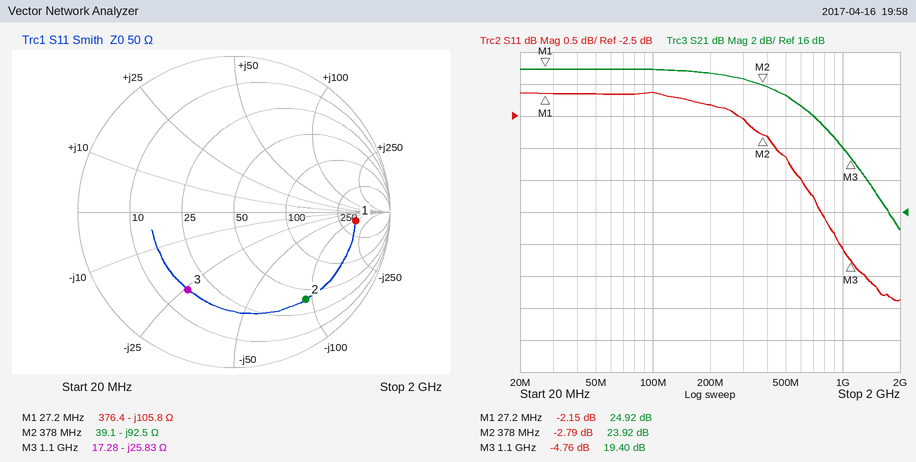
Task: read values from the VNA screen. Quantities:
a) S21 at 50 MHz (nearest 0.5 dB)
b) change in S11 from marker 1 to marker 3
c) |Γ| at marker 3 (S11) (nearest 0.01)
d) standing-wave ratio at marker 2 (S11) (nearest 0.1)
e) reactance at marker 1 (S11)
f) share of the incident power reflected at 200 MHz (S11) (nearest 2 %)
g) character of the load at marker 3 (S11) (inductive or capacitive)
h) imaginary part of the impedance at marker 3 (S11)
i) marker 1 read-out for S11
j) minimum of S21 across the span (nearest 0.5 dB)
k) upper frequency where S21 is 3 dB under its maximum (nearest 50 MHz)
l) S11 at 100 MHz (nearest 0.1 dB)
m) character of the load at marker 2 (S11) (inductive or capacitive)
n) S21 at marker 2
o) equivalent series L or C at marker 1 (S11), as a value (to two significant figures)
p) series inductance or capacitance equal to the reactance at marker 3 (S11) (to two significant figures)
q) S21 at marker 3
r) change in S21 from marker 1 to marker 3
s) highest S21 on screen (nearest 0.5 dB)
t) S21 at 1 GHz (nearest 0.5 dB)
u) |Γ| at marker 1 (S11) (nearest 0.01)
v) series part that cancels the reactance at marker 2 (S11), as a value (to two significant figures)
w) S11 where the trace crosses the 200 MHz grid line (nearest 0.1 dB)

25.0 dB
-2.61 dB
0.58
6.3
-105.8 Ω
58 %
capacitive
-25.83 Ω
-2.15 dB
15.0 dB
700 MHz
-2.1 dB
capacitive
23.92 dB
55 pF
5.6 pF
19.40 dB
-5.52 dB
25.0 dB
20.0 dB
0.78
39 nH
-2.3 dB
